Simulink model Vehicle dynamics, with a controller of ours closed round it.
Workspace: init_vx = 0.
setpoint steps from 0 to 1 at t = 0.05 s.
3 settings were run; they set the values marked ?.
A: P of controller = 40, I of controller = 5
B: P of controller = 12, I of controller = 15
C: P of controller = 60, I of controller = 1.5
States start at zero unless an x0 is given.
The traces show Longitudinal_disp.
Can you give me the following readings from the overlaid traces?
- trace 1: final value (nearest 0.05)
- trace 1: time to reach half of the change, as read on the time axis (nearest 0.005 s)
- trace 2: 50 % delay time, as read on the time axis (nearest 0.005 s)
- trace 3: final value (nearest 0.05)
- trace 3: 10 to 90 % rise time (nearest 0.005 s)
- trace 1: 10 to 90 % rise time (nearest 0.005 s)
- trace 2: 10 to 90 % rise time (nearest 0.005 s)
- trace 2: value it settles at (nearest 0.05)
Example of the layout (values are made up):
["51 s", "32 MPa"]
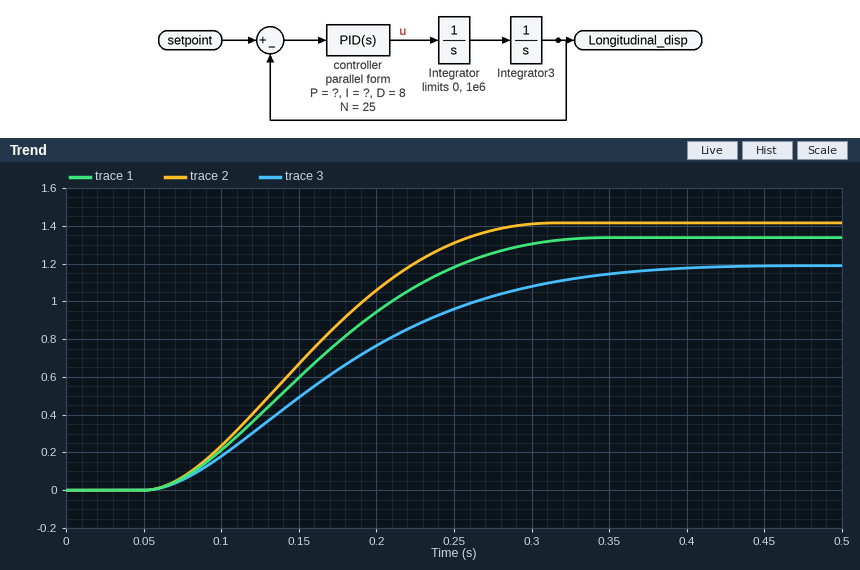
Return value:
["1.35", "0.160 s", "0.155 s", "1.20", "0.205 s", "0.170 s", "0.155 s", "1.40"]
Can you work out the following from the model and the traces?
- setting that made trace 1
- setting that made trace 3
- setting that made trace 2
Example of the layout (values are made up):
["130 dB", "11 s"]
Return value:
["A", "B", "C"]
